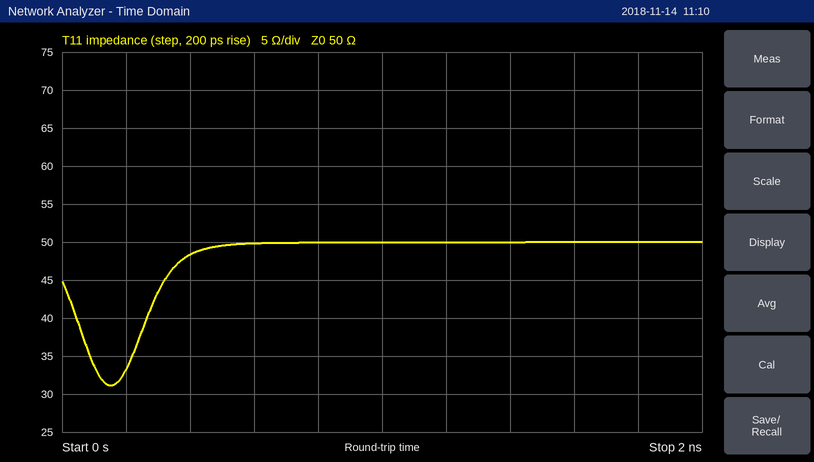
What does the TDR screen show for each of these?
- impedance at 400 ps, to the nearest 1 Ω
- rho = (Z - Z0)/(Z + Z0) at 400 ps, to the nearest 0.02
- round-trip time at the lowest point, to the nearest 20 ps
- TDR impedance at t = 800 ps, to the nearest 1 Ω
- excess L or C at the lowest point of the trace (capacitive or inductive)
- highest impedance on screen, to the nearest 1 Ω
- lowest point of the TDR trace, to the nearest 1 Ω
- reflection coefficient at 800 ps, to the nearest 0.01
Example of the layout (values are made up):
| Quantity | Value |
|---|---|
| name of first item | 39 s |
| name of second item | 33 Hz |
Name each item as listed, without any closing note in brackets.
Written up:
| Quantity | Value |
|---|---|
| impedance at 400 ps, to the nearest 1 Ω | 48 Ω |
| rho = (Z - Z0)/(Z + Z0) at 400 ps, to the nearest 0.02 | -0.02 |
| round-trip time at the lowest point, to the nearest 20 ps | 160 ps |
| TDR impedance at t = 800 ps, to the nearest 1 Ω | 50 Ω |
| excess L or C at the lowest point of the trace | capacitive |
| highest impedance on screen, to the nearest 1 Ω | 50 Ω |
| lowest point of the TDR trace, to the nearest 1 Ω | 31 Ω |
| reflection coefficient at 800 ps, to the nearest 0.01 | 0.00 |
